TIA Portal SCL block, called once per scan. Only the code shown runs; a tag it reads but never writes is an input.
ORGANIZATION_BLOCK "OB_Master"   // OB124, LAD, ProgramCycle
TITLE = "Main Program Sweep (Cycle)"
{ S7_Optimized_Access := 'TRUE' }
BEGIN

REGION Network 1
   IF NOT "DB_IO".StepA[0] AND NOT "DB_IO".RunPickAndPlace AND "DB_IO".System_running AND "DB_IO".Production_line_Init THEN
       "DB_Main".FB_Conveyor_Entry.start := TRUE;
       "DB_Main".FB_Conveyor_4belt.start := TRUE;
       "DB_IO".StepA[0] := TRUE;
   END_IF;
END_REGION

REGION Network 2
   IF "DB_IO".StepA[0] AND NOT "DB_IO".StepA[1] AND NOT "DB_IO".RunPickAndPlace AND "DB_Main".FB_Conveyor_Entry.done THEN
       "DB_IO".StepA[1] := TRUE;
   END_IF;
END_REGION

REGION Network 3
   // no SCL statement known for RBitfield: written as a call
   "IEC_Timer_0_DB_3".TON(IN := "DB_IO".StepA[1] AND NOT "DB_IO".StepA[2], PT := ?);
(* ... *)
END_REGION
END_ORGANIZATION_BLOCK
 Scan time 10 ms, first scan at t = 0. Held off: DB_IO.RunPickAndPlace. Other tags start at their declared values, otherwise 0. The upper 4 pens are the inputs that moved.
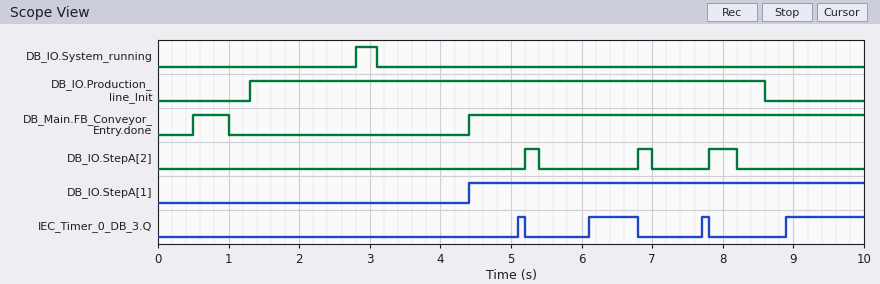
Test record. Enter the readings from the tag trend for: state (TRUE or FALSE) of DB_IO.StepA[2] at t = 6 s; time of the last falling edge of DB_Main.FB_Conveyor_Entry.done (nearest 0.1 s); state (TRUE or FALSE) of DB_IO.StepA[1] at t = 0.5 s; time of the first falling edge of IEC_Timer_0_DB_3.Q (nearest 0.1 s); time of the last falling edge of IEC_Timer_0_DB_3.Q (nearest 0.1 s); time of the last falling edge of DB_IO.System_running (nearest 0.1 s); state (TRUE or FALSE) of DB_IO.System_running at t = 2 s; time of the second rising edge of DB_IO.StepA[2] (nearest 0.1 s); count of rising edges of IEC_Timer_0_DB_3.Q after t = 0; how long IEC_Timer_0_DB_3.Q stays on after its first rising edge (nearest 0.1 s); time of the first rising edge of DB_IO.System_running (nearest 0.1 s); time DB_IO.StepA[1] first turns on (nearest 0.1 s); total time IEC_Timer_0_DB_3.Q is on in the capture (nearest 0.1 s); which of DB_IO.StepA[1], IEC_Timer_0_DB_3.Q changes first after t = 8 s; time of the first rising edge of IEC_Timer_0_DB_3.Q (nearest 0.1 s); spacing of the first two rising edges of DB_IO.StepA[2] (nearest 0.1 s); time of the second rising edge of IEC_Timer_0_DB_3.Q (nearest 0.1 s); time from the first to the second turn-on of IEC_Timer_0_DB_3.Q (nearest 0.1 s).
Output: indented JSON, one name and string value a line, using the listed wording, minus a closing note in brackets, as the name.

{
  "state (TRUE or FALSE) of DB_IO.StepA[2] at t = 6 s": "FALSE",
  "time of the last falling edge of DB_Main.FB_Conveyor_Entry.done": "1.0 s",
  "state (TRUE or FALSE) of DB_IO.StepA[1] at t = 0.5 s": "FALSE",
  "time of the first falling edge of IEC_Timer_0_DB_3.Q": "5.2 s",
  "time of the last falling edge of IEC_Timer_0_DB_3.Q": "7.8 s",
  "time of the last falling edge of DB_IO.System_running": "3.1 s",
  "state (TRUE or FALSE) of DB_IO.System_running at t = 2 s": "FALSE",
  "time of the second rising edge of DB_IO.StepA[2]": "6.8 s",
  "count of rising edges of IEC_Timer_0_DB_3.Q after t = 0": "4",
  "how long IEC_Timer_0_DB_3.Q stays on after its first rising edge": "0.1 s",
  "time of the first rising edge of DB_IO.System_running": "2.8 s",
  "time DB_IO.StepA[1] first turns on": "4.4 s",
  "total time IEC_Timer_0_DB_3.Q is on in the capture": "2.0 s",
  "which of DB_IO.StepA[1], IEC_Timer_0_DB_3.Q changes first after t = 8 s": "IEC_Timer_0_DB_3.Q",
  "time of the first rising edge of IEC_Timer_0_DB_3.Q": "5.1 s",
  "spacing of the first two rising edges of DB_IO.StepA[2]": "1.6 s",
  "time of the second rising edge of IEC_Timer_0_DB_3.Q": "6.1 s",
  "time from the first to the second turn-on of IEC_Timer_0_DB_3.Q": "1.0 s"
}
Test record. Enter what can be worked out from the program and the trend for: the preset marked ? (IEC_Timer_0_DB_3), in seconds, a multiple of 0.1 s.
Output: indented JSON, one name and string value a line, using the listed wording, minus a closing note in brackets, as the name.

{
  "the preset marked ? (IEC_Timer_0_DB_3), in seconds, a multiple of 0.1 s": "0.7 s"
}
